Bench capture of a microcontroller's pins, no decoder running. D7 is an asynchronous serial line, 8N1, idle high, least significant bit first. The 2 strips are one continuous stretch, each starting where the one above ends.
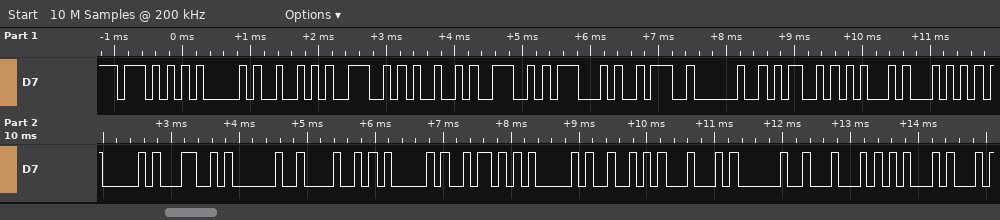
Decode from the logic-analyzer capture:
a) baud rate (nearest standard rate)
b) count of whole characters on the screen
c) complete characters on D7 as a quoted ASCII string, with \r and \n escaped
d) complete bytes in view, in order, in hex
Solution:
9600 baud
24
"WARNING: METAL HAZARD DE"
0x57 0x41 0x52 0x4E 0x49 0x4E 0x47 0x3A 0x20 0x4D 0x45 0x54 0x41 0x4C 0x20 0x48 0x41 0x5A 0x41 0x52 0x44 0x20 0x44 0x45
